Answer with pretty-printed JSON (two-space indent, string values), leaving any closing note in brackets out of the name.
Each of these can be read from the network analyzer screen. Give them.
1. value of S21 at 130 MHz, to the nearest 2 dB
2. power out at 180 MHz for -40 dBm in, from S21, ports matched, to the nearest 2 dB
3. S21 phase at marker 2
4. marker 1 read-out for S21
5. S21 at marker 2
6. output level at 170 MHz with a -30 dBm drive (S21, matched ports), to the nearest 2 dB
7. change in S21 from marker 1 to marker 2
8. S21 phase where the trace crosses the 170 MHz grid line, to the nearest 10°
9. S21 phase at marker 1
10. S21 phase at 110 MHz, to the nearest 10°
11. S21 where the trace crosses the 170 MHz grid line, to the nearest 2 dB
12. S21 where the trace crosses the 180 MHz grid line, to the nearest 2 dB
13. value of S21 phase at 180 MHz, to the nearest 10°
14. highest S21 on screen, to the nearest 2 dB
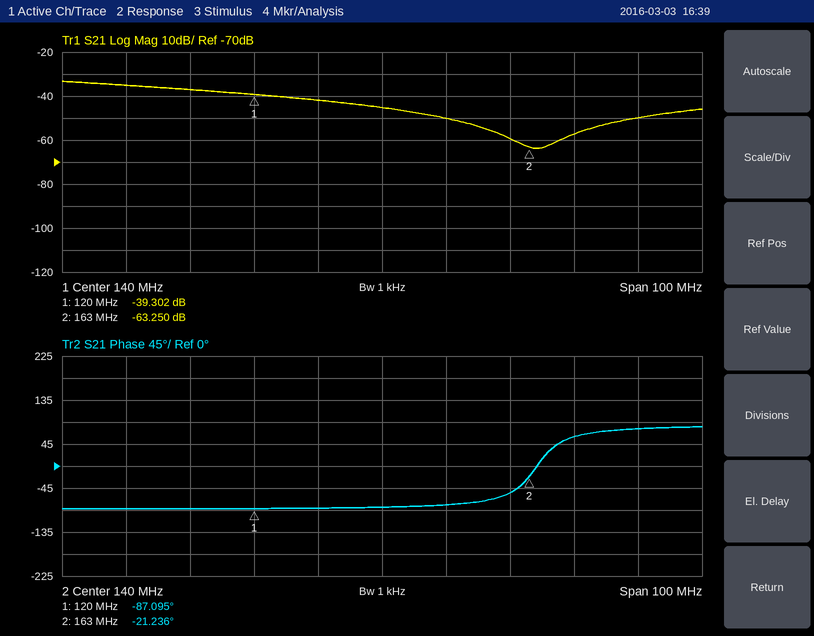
{
  "value of S21 at 130 MHz, to the nearest 2 dB": "-42 dB",
  "power out at 180 MHz for -40 dBm in, from S21, ports matched, to the nearest 2 dB": "-90 dBm",
  "S21 phase at marker 2": "-21.236°",
  "marker 1 read-out for S21": "-39.302 dB",
  "S21 at marker 2": "-63.250 dB",
  "output level at 170 MHz with a -30 dBm drive (S21, matched ports), to the nearest 2 dB": "-88 dBm",
  "change in S21 from marker 1 to marker 2": "-23.948 dB",
  "S21 phase where the trace crosses the 170 MHz grid line, to the nearest 10°": "60°",
  "S21 phase at marker 1": "-87.095°",
  "S21 phase at 110 MHz, to the nearest 10°": "-90°",
  "S21 where the trace crosses the 170 MHz grid line, to the nearest 2 dB": "-58 dB",
  "S21 where the trace crosses the 180 MHz grid line, to the nearest 2 dB": "-50 dB",
  "value of S21 phase at 180 MHz, to the nearest 10°": "80°",
  "highest S21 on screen, to the nearest 2 dB": "-34 dB"
}
